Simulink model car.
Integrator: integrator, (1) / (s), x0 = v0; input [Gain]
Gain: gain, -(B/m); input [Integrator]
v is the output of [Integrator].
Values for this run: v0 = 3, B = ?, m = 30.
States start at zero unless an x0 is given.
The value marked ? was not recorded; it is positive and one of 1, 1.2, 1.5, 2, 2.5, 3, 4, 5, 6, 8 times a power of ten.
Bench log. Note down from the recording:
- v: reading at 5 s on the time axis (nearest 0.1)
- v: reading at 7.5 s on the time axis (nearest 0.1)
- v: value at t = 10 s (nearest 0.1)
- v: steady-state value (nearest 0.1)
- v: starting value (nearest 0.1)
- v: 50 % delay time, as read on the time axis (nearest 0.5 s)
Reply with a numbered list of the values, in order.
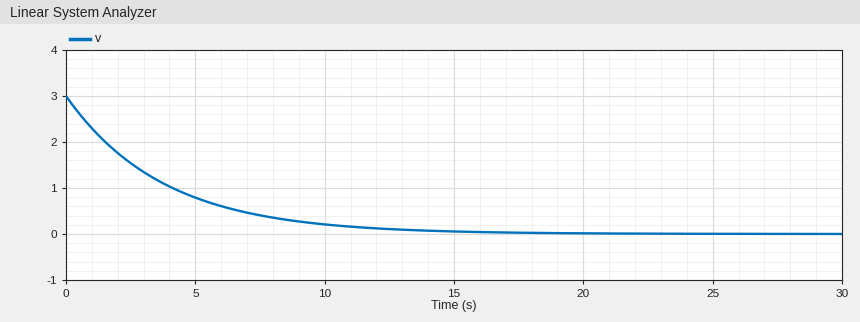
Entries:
1. 0.8
2. 0.4
3. 0.2
4. 0.0
5. 3.0
6. 2.5 s
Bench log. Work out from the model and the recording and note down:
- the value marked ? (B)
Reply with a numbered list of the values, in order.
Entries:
1. 8
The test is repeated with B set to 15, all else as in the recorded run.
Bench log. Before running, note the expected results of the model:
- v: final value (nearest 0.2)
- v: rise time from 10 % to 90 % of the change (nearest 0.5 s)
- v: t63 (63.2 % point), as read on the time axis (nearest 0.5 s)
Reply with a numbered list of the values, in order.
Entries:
1. 0.0
2. 4.5 s
3. 2.0 s
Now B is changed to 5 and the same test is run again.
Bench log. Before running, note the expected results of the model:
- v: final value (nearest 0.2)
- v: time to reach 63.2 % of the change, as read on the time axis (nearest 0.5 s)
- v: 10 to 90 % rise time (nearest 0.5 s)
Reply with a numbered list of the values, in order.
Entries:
1. 0.0
2. 6.0 s
3. 13.0 s
